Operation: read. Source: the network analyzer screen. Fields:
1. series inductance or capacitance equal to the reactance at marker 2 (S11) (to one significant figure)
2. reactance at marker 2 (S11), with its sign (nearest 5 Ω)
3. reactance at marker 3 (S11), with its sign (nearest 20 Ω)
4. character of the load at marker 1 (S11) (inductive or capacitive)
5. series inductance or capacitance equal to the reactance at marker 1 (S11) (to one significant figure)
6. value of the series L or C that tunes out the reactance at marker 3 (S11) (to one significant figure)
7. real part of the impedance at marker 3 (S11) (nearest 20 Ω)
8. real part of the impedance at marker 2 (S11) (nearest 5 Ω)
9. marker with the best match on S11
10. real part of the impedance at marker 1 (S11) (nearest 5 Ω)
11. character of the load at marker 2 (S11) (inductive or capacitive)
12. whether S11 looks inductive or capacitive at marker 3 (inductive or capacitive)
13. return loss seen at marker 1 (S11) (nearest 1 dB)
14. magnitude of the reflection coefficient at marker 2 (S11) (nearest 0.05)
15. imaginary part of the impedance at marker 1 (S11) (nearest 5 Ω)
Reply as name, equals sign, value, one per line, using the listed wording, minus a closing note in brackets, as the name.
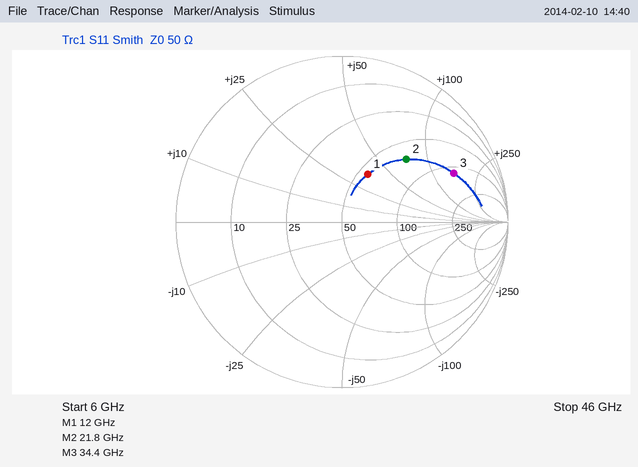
series inductance or capacitance equal to the reactance at marker 2 (S11) = 500 pH
reactance at marker 2 (S11), with its sign = +75 Ω
reactance at marker 3 (S11), with its sign = +160 Ω
character of the load at marker 1 (S11) = inductive
series inductance or capacitance equal to the reactance at marker 1 (S11) = 500 pH
value of the series L or C that tunes out the reactance at marker 3 (S11) = 30 fF
real part of the impedance at marker 3 (S11) = 120 Ω
real part of the impedance at marker 2 (S11) = 70 Ω
marker with the best match on S11 = marker 1
real part of the impedance at marker 1 (S11) = 55 Ω
character of the load at marker 2 (S11) = inductive
whether S11 looks inductive or capacitive at marker 3 = inductive
return loss seen at marker 1 (S11) = 10 dB
magnitude of the reflection coefficient at marker 2 (S11) = 0.55
imaginary part of the impedance at marker 1 (S11) = +35 Ω
